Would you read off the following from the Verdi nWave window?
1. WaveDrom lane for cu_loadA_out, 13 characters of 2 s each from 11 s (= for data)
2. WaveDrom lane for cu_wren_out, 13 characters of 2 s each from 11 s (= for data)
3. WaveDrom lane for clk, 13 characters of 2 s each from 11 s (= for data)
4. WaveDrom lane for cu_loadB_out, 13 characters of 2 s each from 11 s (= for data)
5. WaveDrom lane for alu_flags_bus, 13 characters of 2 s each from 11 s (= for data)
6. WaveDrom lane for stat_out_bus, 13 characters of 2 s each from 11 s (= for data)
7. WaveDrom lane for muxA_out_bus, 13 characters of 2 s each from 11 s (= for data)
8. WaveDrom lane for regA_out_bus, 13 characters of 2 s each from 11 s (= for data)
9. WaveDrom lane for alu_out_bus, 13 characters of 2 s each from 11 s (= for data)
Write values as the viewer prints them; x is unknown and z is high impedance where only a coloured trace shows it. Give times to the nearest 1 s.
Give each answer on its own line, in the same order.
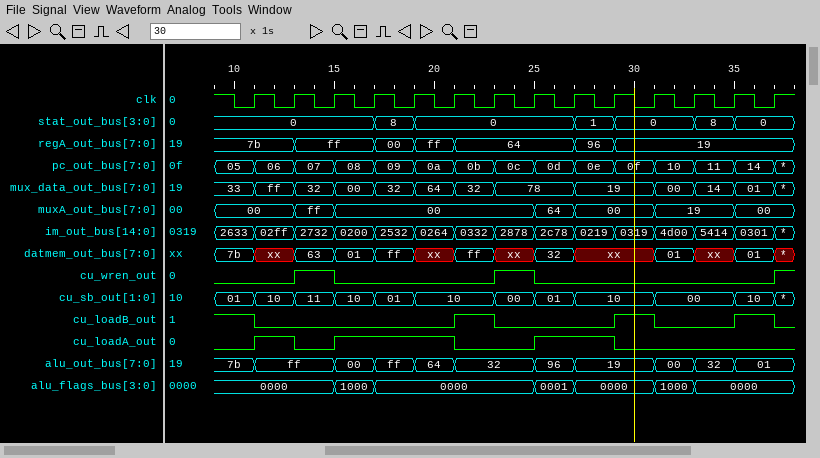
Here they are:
{name: 'cu_loadA_out', wave: '101..0.1.0...'}
{name: 'cu_wren_out', wave: '010...10.....'}
{name: 'clk', wave: 'p............'}
{name: 'cu_loadB_out', wave: '0....10..10.1'}
{name: 'alu_flags_bus', wave: '=.==...==.==.', data: '0000 1000 0000 0001 0000 1000 0000'}
{name: 'stat_out_bus', wave: '=..==...==.==', data: '0 8 0 1 0 8 0'}
{name: 'muxA_out_bus', wave: '===....==.=.=', data: '00 ff 00 64 00 19 00'}
{name: 'regA_out_bus', wave: '==.===..==...', data: '7b ff 00 ff 64 96 19'}
{name: 'alu_out_bus', wave: '=.====.==.===', data: 'ff 00 ff 64 32 96 19 00 32 01'}
